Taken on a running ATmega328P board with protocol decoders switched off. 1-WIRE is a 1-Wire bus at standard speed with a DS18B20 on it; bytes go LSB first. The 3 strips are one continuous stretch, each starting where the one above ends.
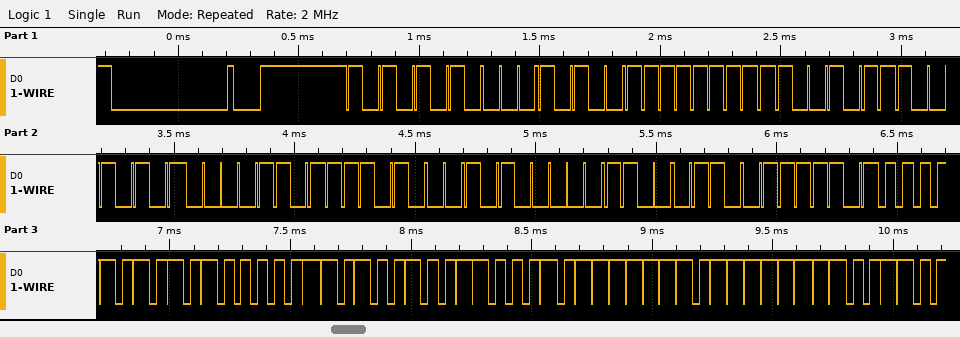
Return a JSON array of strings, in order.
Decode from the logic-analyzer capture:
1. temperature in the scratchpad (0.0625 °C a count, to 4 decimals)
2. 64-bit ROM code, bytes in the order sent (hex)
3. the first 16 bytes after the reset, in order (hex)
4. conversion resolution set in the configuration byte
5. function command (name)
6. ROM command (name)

["85.0000 °C", "28 FF D3 A9 B0 17 05 63", "55 28 FF D3 A9 B0 17 05 63 BE 50 05 4B 46 7F FF", "12 bits", "Read Scratchpad", "Match ROM"]
